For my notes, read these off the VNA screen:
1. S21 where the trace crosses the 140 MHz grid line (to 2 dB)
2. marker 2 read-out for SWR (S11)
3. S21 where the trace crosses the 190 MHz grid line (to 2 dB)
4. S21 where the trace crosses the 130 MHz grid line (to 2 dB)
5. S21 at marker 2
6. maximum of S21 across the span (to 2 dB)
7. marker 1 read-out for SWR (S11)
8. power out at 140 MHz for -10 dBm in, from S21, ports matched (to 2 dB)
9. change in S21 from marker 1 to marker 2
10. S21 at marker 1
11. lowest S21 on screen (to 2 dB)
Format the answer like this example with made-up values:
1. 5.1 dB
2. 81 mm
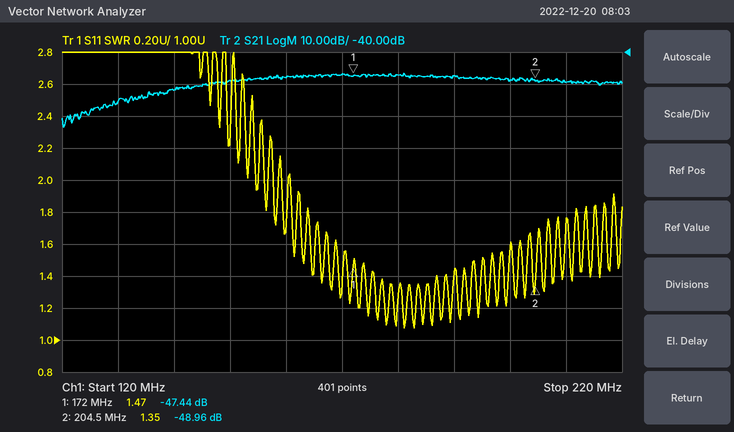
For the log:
1. -52 dB
2. 1.35
3. -48 dB
4. -56 dB
5. -48.96 dB
6. -46 dB
7. 1.47
8. -62 dBm
9. -1.52 dB
10. -47.44 dB
11. -64 dB
